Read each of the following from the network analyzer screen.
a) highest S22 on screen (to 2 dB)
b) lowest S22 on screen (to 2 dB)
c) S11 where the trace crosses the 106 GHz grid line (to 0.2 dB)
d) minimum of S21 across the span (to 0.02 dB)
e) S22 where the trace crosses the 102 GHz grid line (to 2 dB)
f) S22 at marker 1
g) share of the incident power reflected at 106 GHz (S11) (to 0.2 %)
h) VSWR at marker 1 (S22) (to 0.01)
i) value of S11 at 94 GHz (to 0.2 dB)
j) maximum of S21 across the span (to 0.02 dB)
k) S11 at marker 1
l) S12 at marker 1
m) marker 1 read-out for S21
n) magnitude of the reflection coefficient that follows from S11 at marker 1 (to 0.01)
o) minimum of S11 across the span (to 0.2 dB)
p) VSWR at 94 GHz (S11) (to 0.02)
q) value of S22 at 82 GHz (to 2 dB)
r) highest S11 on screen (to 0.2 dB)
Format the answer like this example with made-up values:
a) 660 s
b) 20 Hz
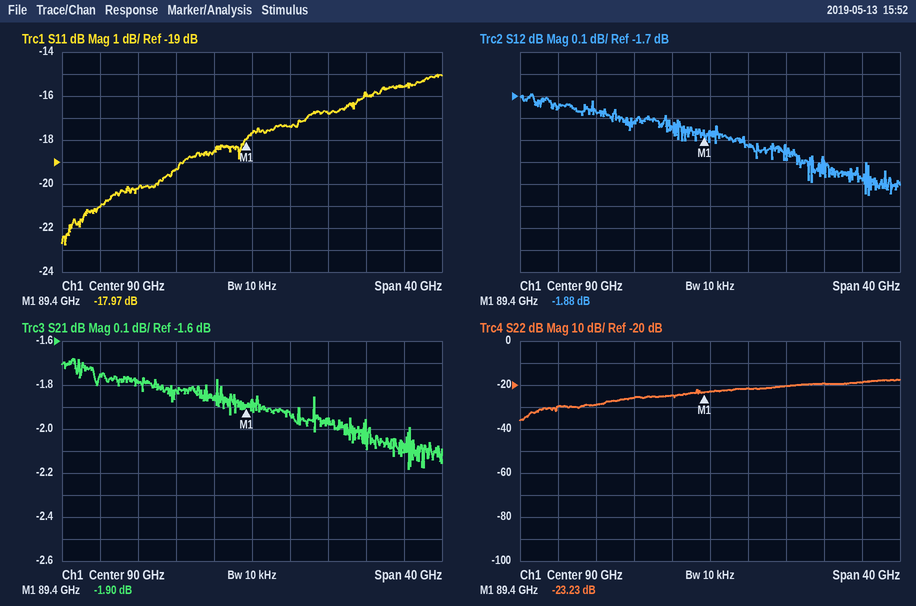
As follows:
a) -18 dB
b) -36 dB
c) -15.6 dB
d) -2.18 dB
e) -20 dB
f) -23.23 dB
g) 2.8 %
h) 1.15
i) -17.4 dB
j) -1.68 dB
k) -17.97 dB
l) -1.88 dB
m) -1.90 dB
n) 0.13
o) -22.8 dB
p) 1.32
q) -26 dB
r) -15.0 dB
